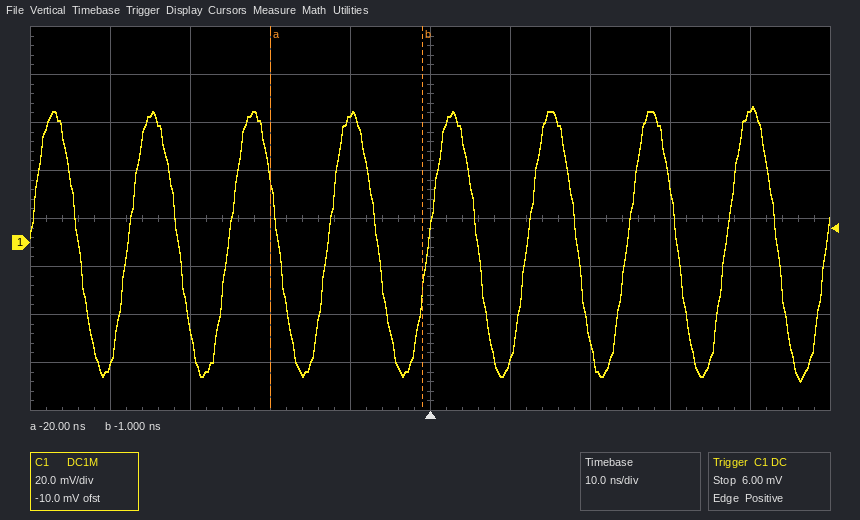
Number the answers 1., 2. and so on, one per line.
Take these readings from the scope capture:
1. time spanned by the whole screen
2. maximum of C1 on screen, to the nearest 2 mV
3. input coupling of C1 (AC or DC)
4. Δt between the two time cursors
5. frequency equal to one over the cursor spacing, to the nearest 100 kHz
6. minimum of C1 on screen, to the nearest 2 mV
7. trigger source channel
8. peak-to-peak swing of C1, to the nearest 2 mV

1. 100 ns
2. 56 mV
3. DC
4. 19 ns
5. 52.6 MHz
6. -58 mV
7. C1
8. 114 mV
